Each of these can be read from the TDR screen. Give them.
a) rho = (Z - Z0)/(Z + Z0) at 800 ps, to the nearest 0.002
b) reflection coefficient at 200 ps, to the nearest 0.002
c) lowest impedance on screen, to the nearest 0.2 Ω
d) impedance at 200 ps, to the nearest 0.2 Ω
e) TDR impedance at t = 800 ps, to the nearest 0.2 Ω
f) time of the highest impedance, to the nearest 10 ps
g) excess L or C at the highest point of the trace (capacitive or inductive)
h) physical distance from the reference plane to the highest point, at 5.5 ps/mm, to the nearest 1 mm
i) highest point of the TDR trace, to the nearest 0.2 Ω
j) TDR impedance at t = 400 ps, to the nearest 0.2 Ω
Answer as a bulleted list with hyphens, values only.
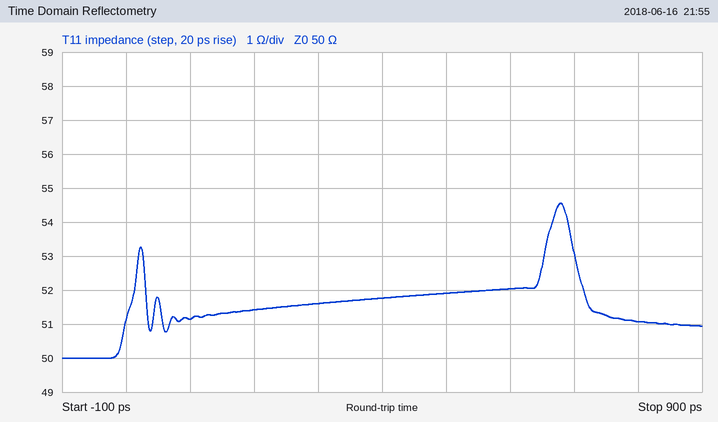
- +0.010
- +0.014
- 50.0 Ω
- 51.4 Ω
- 51.0 Ω
- 680 ps
- inductive
- 62 mm
- 54.6 Ω
- 51.8 Ω
